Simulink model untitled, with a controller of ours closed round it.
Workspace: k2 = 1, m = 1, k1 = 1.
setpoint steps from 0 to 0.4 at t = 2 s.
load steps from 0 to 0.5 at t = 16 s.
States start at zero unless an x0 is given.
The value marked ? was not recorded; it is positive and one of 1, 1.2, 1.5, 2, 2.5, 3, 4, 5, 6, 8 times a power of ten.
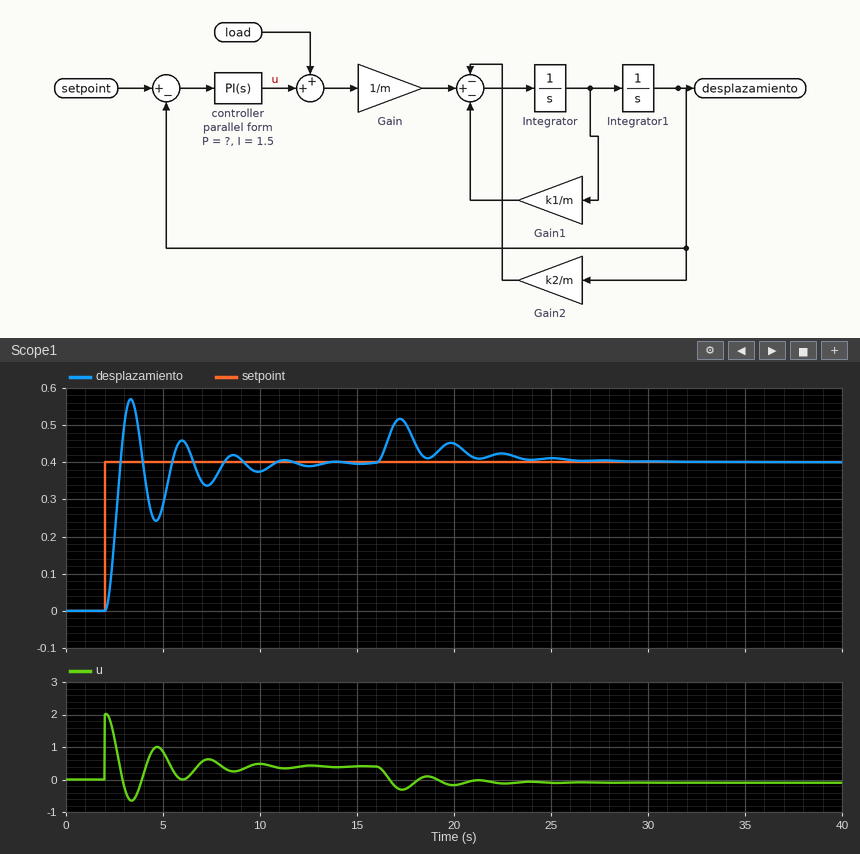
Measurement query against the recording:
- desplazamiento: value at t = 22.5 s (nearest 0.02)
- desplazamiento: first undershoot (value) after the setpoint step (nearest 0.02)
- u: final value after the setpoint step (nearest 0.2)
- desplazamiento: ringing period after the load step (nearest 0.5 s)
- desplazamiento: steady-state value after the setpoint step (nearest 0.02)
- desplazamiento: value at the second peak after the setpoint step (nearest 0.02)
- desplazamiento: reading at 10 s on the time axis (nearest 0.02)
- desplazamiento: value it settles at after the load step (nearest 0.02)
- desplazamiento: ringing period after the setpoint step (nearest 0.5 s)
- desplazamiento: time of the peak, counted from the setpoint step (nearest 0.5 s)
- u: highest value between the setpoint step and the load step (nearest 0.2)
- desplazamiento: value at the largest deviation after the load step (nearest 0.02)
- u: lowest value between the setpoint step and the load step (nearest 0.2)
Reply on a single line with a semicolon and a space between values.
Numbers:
0.42; 0.24; 0.4; 2.5 s; 0.40; 0.46; 0.38; 0.40; 2.5 s; 1.5 s; 2.0; 0.52; -0.6
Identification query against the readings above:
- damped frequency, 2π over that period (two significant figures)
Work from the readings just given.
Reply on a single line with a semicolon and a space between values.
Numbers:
2.5 rad/s
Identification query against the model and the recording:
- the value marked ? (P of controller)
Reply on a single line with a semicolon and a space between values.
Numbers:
5
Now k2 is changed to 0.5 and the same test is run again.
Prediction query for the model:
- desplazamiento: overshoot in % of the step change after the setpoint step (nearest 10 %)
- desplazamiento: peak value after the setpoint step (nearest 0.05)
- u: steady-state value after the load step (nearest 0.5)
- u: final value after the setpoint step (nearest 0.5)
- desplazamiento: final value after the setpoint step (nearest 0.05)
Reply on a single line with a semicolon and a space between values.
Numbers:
50 %; 0.60; -0.5; 0.0; 0.40
